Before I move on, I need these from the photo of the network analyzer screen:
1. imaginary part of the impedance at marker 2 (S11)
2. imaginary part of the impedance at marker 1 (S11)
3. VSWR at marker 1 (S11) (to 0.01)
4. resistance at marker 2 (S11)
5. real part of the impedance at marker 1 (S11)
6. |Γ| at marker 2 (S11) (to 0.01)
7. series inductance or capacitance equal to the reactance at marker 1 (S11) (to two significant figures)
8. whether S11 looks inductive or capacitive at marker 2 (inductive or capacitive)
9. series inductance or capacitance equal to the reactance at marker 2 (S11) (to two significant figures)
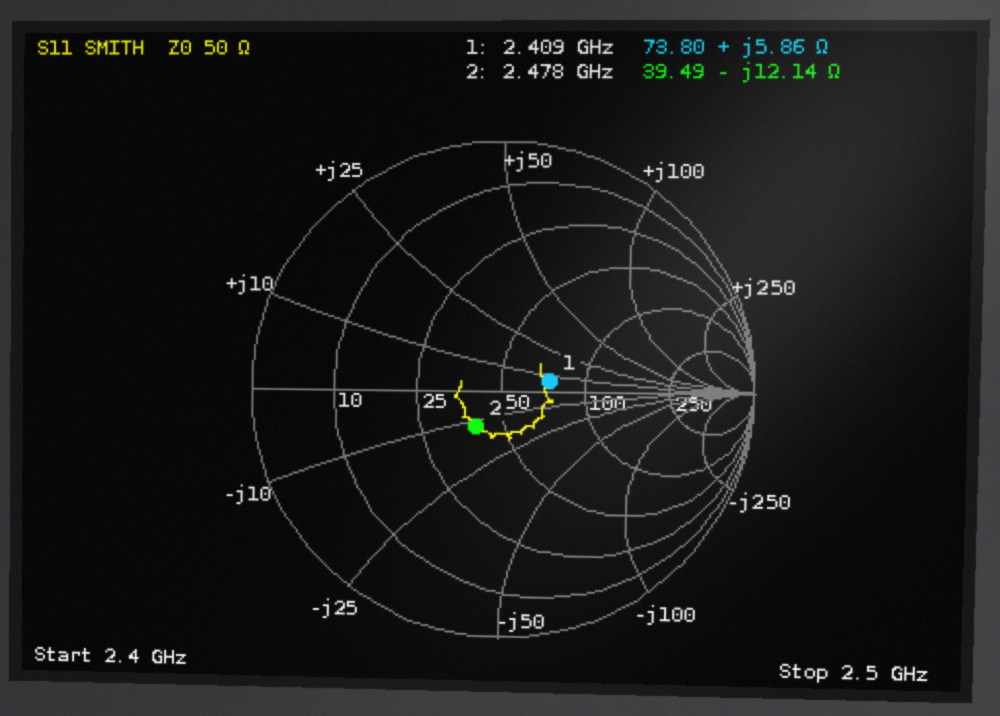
-12.14 Ω
+5.86 Ω
1.49
39.49 Ω
73.80 Ω
0.18
390 pH
capacitive
5.3 pF
